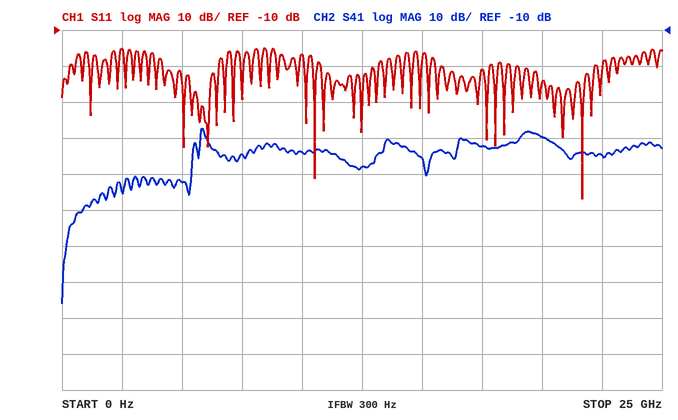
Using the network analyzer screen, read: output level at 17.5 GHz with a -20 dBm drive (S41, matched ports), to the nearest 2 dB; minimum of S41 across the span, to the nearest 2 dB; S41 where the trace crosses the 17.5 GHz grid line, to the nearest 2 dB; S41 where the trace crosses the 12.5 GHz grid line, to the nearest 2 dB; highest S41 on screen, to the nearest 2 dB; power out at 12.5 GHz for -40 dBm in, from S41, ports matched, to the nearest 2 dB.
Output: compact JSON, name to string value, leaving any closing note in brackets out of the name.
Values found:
{"output level at 17.5 GHz with a -20 dBm drive (S41, matched ports), to the nearest 2 dB": "-62 dBm", "minimum of S41 across the span, to the nearest 2 dB": "-86 dB", "S41 where the trace crosses the 17.5 GHz grid line, to the nearest 2 dB": "-42 dB", "S41 where the trace crosses the 12.5 GHz grid line, to the nearest 2 dB": "-48 dB", "highest S41 on screen, to the nearest 2 dB": "-38 dB", "power out at 12.5 GHz for -40 dBm in, from S41, ports matched, to the nearest 2 dB": "-88 dBm"}
